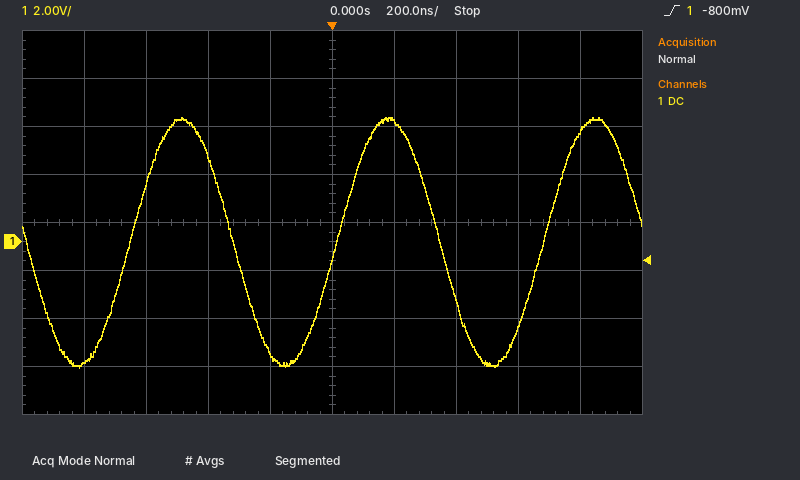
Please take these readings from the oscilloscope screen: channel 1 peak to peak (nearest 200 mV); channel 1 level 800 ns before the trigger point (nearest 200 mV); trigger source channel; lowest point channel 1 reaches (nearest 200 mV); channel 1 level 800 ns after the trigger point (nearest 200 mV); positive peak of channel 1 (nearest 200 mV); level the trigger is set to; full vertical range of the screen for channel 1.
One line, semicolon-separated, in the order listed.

10.4 V; -5.0 V; channel 1; -5.2 V; 4.6 V; 5.2 V; -800 mV; 16 V
